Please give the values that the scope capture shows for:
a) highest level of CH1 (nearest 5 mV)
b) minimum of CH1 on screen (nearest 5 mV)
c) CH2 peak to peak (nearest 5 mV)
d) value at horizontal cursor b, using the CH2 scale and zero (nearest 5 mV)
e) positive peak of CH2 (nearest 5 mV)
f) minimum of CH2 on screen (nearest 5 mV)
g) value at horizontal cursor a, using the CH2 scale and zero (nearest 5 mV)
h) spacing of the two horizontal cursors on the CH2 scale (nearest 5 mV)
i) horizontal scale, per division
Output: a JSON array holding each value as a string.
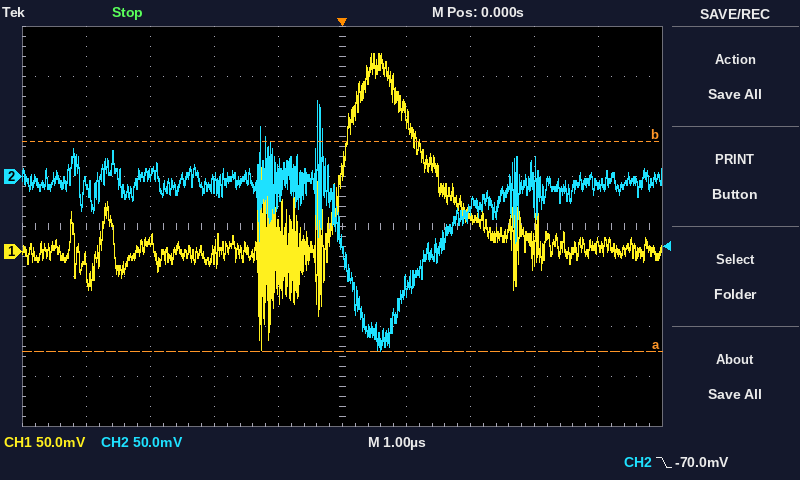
["200 mV", "-100 mV", "250 mV", "35 mV", "75 mV", "-175 mV", "-175 mV", "210 mV", "1 µs"]
